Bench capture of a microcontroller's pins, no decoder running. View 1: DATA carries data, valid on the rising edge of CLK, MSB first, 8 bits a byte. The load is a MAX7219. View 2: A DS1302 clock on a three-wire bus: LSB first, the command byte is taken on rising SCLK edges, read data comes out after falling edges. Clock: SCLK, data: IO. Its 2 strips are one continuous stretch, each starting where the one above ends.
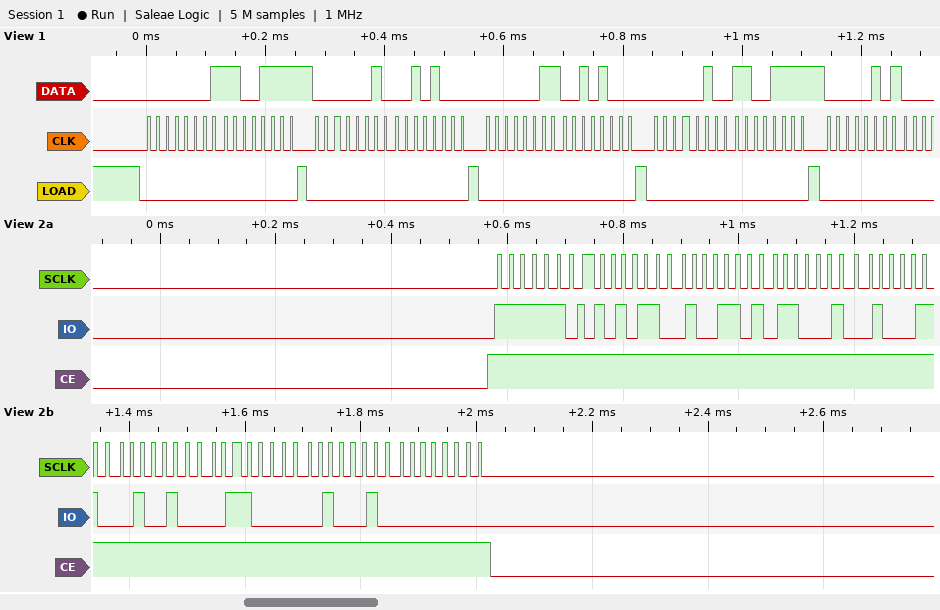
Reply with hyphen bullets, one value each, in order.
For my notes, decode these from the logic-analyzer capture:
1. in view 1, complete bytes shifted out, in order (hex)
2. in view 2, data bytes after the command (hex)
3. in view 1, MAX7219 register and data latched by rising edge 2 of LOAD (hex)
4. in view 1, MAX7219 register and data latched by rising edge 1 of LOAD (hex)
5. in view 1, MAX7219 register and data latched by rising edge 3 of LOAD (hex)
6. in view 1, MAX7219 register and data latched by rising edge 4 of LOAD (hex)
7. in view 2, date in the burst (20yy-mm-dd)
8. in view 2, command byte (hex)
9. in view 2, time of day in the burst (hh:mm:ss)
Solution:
- 01 CF 02 28 03 28 04 CF 05
- 35 59 23 31 12 06 22 00
- register 0x2, data 0x28
- register 0x1, data 0xCF
- register 0x3, data 0x28
- register 0x4, data 0xCF
- 2022-12-31
- 0xBF
- 23:59:35
